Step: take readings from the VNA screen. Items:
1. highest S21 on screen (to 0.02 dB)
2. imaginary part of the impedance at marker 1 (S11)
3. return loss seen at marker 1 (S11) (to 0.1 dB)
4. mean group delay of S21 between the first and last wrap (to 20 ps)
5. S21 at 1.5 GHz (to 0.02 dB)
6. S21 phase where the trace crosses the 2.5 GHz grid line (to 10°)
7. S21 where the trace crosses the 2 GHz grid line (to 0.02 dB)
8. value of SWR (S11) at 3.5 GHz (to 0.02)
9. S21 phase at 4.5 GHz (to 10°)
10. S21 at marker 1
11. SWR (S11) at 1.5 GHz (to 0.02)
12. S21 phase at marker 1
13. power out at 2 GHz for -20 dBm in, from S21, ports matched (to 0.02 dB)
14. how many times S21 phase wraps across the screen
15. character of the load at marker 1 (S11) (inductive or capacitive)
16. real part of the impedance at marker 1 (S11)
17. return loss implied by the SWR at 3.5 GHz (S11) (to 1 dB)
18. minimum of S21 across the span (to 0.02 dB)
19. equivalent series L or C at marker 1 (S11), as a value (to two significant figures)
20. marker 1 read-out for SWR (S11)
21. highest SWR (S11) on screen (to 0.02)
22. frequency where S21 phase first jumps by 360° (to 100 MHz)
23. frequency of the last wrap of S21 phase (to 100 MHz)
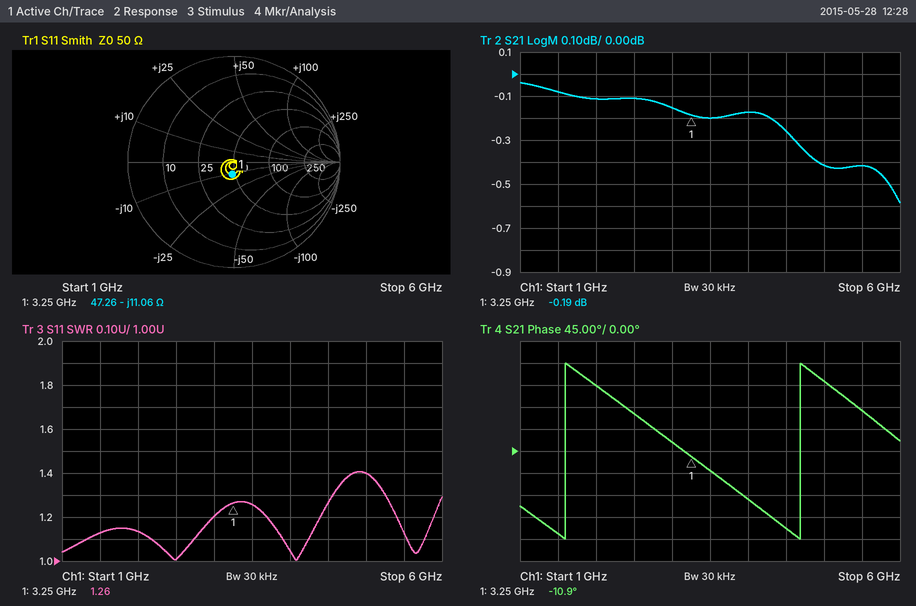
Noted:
-0.04 dB
-11.06 Ω
18.7 dB
320 ps
-0.08 dB
80°
-0.12 dB
1.26
-160°
-0.19 dB
1.12
-10.9°
-20.12 dBm
2
capacitive
47.26 Ω
19 dB
-0.58 dB
4.4 pF
1.26
1.40
1.6 GHz
4.7 GHz
